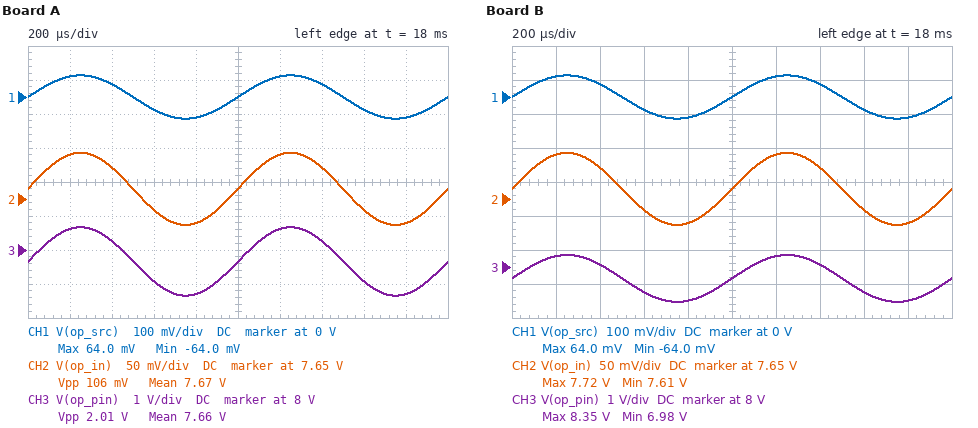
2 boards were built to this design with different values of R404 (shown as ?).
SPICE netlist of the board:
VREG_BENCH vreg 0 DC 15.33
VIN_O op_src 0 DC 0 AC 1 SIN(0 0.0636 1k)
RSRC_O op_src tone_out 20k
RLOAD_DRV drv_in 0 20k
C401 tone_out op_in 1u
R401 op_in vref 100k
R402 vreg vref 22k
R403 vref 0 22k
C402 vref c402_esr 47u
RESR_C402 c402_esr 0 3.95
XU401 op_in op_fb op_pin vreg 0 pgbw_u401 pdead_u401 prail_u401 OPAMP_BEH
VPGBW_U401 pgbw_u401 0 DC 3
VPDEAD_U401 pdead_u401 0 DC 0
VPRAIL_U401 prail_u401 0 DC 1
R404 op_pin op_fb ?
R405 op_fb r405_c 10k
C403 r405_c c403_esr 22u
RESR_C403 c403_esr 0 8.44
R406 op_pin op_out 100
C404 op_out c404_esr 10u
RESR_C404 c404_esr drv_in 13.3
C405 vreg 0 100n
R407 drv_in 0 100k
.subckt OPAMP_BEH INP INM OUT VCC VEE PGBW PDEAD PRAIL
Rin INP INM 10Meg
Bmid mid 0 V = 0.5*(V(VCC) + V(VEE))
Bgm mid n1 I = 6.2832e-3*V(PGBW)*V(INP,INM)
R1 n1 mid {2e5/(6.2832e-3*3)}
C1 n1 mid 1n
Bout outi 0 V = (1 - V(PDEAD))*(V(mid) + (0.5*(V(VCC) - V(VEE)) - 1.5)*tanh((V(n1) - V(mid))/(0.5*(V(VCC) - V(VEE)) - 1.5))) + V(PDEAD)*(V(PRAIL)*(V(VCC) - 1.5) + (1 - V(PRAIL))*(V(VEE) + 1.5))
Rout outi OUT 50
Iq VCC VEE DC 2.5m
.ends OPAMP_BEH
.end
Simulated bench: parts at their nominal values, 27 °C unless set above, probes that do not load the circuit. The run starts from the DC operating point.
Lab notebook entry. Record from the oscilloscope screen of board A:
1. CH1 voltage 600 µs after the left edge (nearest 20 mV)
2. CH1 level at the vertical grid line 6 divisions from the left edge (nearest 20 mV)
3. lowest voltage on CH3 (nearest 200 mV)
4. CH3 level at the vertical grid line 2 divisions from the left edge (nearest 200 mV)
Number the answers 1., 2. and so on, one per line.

1. -40 mV
2. 60 mV
3. 6.6 V
4. 8.2 V
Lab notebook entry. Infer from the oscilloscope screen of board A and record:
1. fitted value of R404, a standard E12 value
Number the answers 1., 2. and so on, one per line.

1. 180 kΩ
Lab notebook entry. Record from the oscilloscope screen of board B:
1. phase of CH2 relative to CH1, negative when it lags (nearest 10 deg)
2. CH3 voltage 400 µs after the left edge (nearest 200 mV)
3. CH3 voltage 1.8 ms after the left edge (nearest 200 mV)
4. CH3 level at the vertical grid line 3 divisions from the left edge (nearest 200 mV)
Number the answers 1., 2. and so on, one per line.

1. 0 deg
2. 8.0 V
3. 7.0 V
4. 7.2 V
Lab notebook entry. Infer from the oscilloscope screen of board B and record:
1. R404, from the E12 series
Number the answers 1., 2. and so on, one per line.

1. 120 kΩ
